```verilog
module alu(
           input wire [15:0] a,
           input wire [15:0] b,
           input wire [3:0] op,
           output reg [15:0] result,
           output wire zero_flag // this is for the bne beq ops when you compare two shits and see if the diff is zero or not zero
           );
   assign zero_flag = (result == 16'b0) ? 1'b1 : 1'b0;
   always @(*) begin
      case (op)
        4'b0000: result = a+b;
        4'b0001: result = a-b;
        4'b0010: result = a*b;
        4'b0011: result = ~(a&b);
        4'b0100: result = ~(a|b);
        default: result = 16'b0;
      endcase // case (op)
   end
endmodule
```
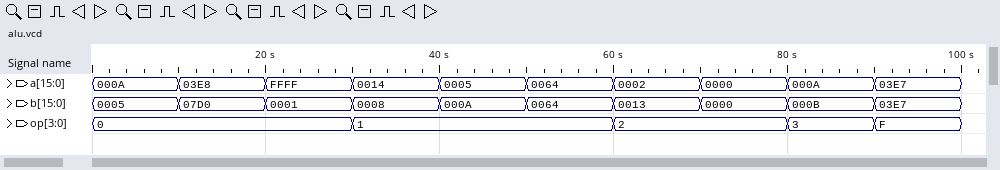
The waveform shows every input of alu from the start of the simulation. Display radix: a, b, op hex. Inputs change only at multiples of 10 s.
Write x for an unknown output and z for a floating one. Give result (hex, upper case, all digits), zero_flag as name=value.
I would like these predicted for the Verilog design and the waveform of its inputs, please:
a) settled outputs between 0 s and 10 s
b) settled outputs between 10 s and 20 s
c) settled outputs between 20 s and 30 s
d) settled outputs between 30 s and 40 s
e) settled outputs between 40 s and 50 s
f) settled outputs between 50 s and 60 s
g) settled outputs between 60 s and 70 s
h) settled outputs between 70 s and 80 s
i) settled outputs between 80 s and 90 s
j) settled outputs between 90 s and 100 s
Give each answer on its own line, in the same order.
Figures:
result=000F, zero_flag=0
result=0BB8, zero_flag=0
result=0000, zero_flag=1
result=000C, zero_flag=0
result=FFFB, zero_flag=0
result=0000, zero_flag=1
result=0026, zero_flag=0
result=0000, zero_flag=1
result=FFF5, zero_flag=0
result=0000, zero_flag=1
